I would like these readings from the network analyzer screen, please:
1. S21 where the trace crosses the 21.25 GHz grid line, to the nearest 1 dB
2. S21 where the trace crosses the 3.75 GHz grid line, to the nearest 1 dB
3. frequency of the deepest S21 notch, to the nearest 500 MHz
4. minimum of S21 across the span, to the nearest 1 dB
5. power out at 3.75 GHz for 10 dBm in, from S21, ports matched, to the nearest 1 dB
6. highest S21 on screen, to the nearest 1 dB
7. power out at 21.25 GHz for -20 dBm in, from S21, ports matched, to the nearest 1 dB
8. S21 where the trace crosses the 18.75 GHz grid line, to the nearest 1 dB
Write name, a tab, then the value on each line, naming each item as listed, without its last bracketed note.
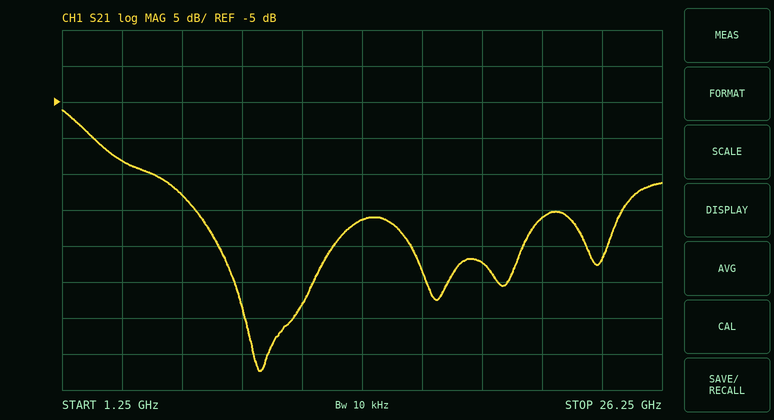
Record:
S21 where the trace crosses the 21.25 GHz grid line, to the nearest 1 dB	-21 dB
S21 where the trace crosses the 3.75 GHz grid line, to the nearest 1 dB	-13 dB
frequency of the deepest S21 notch, to the nearest 500 MHz	9.5 GHz
minimum of S21 across the span, to the nearest 1 dB	-42 dB
power out at 3.75 GHz for 10 dBm in, from S21, ports matched, to the nearest 1 dB	-3 dBm
highest S21 on screen, to the nearest 1 dB	-6 dB
power out at 21.25 GHz for -20 dBm in, from S21, ports matched, to the nearest 1 dB	-41 dBm
S21 where the trace crosses the 18.75 GHz grid line, to the nearest 1 dB	-27 dB
